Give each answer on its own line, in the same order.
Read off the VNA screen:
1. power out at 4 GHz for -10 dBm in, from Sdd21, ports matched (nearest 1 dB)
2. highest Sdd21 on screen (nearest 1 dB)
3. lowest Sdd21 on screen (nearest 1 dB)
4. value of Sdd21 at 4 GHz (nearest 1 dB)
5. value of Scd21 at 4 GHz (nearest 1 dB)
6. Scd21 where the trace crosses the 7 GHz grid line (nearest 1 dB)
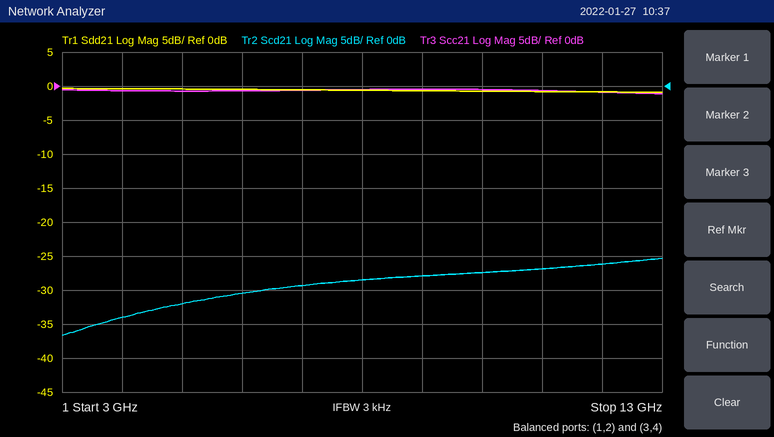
-10 dBm
0 dB
-1 dB
0 dB
-34 dB
-29 dB
